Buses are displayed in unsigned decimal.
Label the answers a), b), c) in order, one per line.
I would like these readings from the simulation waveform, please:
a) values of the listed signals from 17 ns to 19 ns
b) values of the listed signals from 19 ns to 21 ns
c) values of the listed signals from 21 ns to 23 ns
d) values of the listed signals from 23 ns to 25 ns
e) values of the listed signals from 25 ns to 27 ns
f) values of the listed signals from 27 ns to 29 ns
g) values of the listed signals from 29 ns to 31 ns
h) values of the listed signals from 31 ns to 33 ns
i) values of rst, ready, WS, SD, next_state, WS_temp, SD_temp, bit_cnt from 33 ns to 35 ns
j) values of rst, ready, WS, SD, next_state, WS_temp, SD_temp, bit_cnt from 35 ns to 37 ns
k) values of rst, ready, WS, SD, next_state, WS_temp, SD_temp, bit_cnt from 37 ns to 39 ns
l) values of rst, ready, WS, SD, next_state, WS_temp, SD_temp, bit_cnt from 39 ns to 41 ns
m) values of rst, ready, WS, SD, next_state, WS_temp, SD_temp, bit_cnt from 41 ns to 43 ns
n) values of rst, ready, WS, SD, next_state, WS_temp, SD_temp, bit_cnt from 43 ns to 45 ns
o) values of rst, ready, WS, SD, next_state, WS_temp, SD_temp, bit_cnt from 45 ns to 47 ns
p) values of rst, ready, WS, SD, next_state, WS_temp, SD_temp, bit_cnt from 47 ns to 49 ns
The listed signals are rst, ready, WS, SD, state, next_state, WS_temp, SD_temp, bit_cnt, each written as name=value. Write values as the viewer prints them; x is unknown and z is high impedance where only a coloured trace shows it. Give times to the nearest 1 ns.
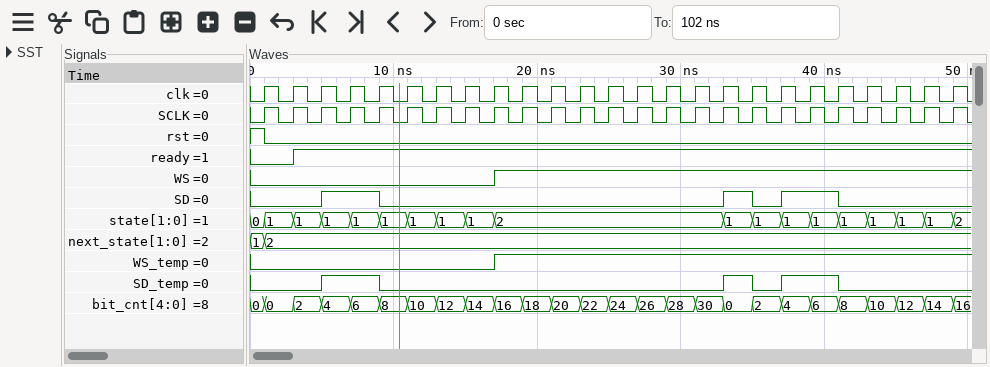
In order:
a) rst=0, ready=1, WS=1, SD=0, state=2, next_state=2, WS_temp=1, SD_temp=0, bit_cnt=16
b) rst=0, ready=1, WS=1, SD=0, state=2, next_state=2, WS_temp=1, SD_temp=0, bit_cnt=18
c) rst=0, ready=1, WS=1, SD=0, state=2, next_state=2, WS_temp=1, SD_temp=0, bit_cnt=20
d) rst=0, ready=1, WS=1, SD=0, state=2, next_state=2, WS_temp=1, SD_temp=0, bit_cnt=22
e) rst=0, ready=1, WS=1, SD=0, state=2, next_state=2, WS_temp=1, SD_temp=0, bit_cnt=24
f) rst=0, ready=1, WS=1, SD=0, state=2, next_state=2, WS_temp=1, SD_temp=0, bit_cnt=26
g) rst=0, ready=1, WS=1, SD=0, state=2, next_state=2, WS_temp=1, SD_temp=0, bit_cnt=28
h) rst=0, ready=1, WS=1, SD=0, state=2, next_state=2, WS_temp=1, SD_temp=0, bit_cnt=30
i) rst=0, ready=1, WS=1, SD=1, next_state=2, WS_temp=1, SD_temp=1, bit_cnt=0
j) rst=0, ready=1, WS=1, SD=0, next_state=2, WS_temp=1, SD_temp=0, bit_cnt=2
k) rst=0, ready=1, WS=1, SD=1, next_state=2, WS_temp=1, SD_temp=1, bit_cnt=4
l) rst=0, ready=1, WS=1, SD=1, next_state=2, WS_temp=1, SD_temp=1, bit_cnt=6
m) rst=0, ready=1, WS=1, SD=0, next_state=2, WS_temp=1, SD_temp=0, bit_cnt=8
n) rst=0, ready=1, WS=1, SD=0, next_state=2, WS_temp=1, SD_temp=0, bit_cnt=10
o) rst=0, ready=1, WS=1, SD=0, next_state=2, WS_temp=1, SD_temp=0, bit_cnt=12
p) rst=0, ready=1, WS=1, SD=0, next_state=2, WS_temp=1, SD_temp=0, bit_cnt=14
